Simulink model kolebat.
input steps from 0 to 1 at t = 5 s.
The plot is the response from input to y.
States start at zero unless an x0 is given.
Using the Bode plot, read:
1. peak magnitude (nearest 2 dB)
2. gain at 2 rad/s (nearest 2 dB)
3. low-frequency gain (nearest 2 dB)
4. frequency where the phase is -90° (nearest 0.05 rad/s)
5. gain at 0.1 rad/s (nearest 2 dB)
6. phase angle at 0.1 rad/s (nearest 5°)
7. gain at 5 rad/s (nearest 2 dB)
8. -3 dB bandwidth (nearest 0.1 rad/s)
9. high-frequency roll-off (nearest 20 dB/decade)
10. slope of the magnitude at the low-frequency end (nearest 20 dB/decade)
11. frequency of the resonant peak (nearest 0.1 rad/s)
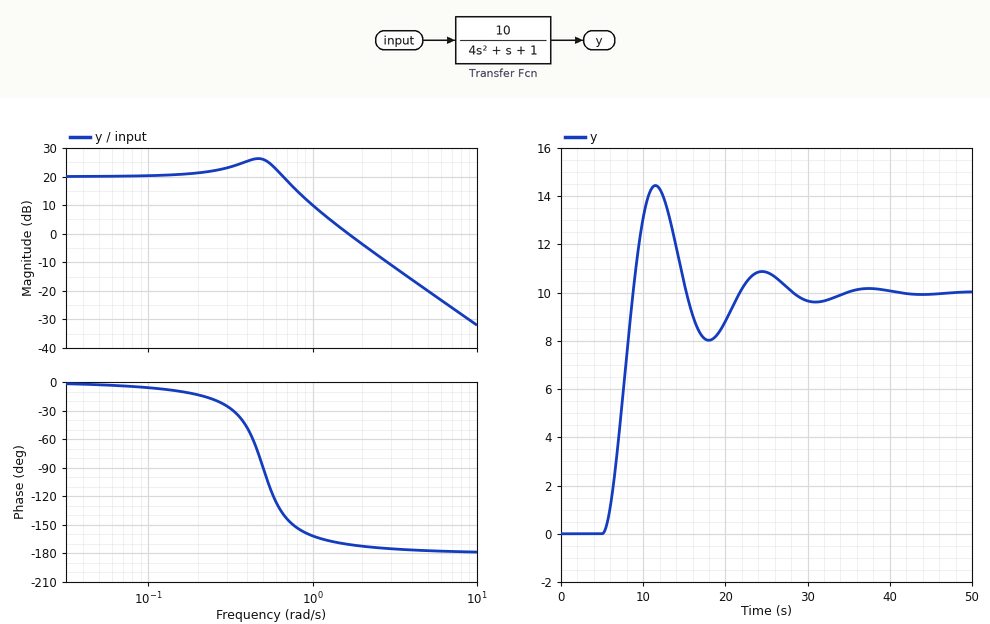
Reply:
26 dB
-4 dB
20 dB
0.50 rad/s
20 dB
-5°
-20 dB
0.7 rad/s
-40 dB/decade
0 dB/decade
0.5 rad/s
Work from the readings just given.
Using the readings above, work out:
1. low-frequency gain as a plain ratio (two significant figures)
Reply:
10
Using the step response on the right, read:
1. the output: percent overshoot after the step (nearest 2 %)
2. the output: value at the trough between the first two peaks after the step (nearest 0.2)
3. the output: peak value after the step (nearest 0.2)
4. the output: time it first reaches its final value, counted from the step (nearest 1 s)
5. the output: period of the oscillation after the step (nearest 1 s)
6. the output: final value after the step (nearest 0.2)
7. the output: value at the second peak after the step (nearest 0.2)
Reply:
44 %
8.0
14.4
4 s
13 s
10.0
10.8
